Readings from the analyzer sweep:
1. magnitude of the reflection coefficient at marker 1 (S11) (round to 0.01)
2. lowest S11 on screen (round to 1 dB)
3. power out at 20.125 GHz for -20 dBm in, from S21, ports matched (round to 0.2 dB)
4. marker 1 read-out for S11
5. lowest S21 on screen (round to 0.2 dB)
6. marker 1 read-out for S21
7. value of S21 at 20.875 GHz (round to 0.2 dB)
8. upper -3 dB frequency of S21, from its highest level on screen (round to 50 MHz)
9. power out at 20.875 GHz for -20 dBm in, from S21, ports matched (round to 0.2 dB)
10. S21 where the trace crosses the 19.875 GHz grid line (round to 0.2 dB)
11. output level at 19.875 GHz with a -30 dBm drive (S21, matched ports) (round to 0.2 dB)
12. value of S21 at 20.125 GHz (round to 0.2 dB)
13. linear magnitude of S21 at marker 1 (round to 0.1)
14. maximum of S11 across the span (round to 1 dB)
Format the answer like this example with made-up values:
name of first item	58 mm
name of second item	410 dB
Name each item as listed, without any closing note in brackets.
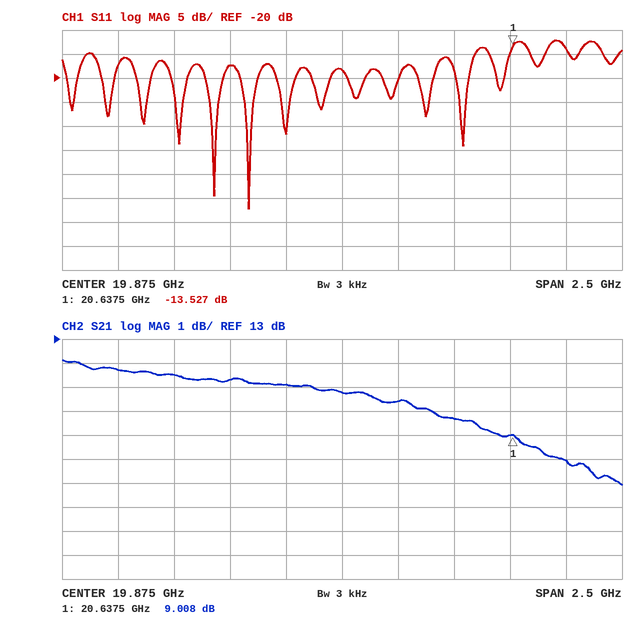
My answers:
magnitude of the reflection coefficient at marker 1 (S11)	0.21
lowest S11 on screen	-47 dB
power out at 20.125 GHz for -20 dBm in, from S21, ports matched	-9.6 dBm
marker 1 read-out for S11	-13.527 dB
lowest S21 on screen	7.0 dB
marker 1 read-out for S21	9.008 dB
value of S21 at 20.875 GHz	8.0 dB
upper -3 dB frequency of S21, from its highest level on screen	20.55 GHz
power out at 20.875 GHz for -20 dBm in, from S21, ports matched	-12.0 dBm
S21 where the trace crosses the 19.875 GHz grid line	10.8 dB
output level at 19.875 GHz with a -30 dBm drive (S21, matched ports)	-19.2 dBm
value of S21 at 20.125 GHz	10.4 dB
linear magnitude of S21 at marker 1	2.8
maximum of S11 across the span	-12 dB
